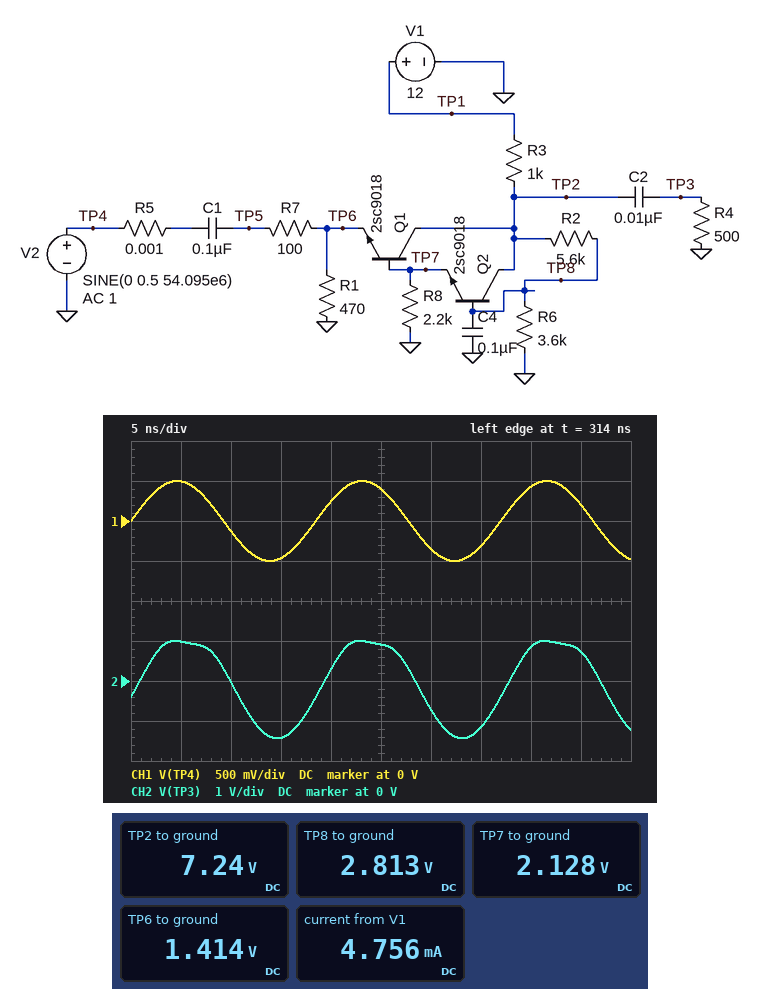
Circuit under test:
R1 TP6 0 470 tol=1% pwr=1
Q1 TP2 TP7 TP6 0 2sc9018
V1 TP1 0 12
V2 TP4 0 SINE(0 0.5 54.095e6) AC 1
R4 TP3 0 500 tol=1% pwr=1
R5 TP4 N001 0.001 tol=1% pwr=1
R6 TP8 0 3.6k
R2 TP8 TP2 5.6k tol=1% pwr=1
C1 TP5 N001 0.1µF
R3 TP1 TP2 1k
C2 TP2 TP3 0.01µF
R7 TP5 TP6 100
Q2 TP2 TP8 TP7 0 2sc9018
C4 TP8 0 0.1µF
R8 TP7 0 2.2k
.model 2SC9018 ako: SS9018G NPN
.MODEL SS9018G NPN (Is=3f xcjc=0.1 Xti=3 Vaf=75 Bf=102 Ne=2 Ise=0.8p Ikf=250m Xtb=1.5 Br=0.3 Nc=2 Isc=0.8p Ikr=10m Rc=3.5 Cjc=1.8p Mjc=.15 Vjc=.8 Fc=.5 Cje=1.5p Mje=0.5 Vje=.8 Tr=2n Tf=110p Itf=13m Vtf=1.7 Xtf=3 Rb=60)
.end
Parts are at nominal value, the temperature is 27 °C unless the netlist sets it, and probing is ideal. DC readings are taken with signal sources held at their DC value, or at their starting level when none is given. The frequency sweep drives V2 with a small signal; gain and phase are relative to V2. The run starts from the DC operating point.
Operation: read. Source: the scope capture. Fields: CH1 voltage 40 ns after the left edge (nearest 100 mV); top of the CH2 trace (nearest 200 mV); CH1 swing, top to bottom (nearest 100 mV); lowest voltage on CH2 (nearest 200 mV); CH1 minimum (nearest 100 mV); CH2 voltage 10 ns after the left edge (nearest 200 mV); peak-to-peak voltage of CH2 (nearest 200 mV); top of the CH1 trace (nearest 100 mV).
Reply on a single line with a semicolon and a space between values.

400 mV; 1.0 V; 1.0 V; -1.4 V; -500 mV; 0 V; 2.4 V; 500 mV
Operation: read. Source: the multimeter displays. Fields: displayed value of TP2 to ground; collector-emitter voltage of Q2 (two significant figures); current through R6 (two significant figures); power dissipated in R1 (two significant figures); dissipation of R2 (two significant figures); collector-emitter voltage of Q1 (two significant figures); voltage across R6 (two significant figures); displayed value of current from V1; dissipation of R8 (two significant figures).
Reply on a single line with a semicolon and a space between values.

7.24 V; 5.1 V; 780 µA; 4.3 mW; 3.5 mW; 5.8 V; 2.8 V; 4.756 mA; 2.1 mW
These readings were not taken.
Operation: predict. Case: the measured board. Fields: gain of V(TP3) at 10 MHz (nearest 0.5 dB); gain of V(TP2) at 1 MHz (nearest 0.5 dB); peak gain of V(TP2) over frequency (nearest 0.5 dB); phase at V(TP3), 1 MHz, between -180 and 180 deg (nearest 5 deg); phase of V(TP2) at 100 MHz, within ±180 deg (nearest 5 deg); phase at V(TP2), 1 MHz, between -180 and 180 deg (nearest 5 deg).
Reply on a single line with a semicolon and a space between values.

9.0 dB; 9.0 dB; 11.5 dB; 0 deg; -25 deg; 0 deg
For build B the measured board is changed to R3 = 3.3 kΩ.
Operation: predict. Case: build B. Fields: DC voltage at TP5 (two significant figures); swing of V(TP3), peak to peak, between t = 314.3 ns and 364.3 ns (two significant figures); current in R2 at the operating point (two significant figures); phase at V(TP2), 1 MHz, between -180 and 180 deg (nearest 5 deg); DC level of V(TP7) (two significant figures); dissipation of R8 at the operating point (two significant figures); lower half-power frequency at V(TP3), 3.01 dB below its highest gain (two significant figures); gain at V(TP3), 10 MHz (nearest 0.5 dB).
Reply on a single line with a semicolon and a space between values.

520 mV; 2.3 V; 530 µA; 0 deg; 1.2 V; 660 µW; 15 kHz; 10.0 dB
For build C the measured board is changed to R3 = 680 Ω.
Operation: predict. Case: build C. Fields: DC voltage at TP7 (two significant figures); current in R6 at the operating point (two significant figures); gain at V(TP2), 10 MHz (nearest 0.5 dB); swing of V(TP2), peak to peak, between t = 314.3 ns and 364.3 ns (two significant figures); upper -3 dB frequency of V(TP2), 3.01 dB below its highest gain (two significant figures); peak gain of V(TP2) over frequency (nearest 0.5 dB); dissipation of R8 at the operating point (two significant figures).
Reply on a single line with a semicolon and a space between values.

2.5 V; 880 µA; 8.0 dB; 2.3 V; 220 MHz; 9.5 dB; 2.8 mW
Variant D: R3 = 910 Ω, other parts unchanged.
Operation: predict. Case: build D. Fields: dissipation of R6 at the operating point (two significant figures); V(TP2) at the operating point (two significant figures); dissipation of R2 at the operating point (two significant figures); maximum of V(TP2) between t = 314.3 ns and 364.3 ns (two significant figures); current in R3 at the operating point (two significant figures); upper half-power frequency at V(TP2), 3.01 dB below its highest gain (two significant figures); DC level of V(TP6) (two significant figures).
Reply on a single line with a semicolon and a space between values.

2.3 mW; 7.5 V; 3.7 mW; 8.5 V; 5.0 mA; 150 MHz; 1.5 V
